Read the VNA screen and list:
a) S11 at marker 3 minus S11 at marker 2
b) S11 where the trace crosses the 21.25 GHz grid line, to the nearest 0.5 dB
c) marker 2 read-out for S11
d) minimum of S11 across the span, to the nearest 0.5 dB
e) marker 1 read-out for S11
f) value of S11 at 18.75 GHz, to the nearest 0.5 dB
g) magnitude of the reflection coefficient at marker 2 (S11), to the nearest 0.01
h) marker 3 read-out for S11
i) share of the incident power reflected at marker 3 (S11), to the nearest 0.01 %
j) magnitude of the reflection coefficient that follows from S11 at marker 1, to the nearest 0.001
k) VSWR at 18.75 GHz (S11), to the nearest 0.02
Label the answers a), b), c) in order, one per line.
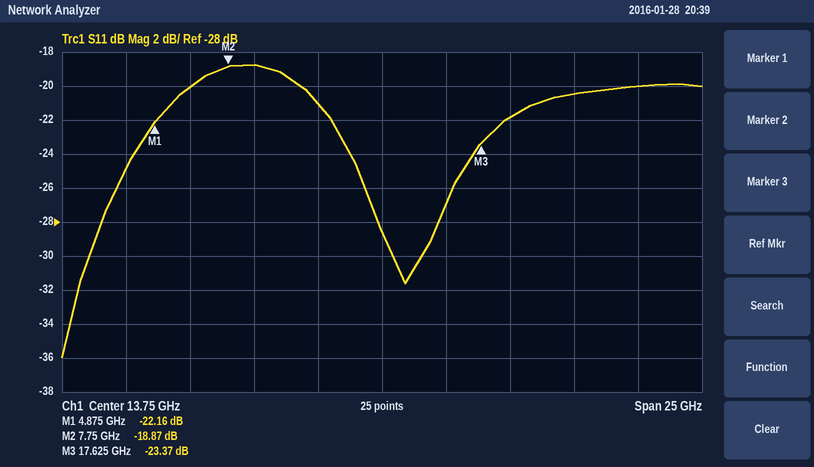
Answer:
a) -4.50 dB
b) -20.5 dB
c) -18.87 dB
d) -36.0 dB
e) -22.16 dB
f) -22.0 dB
g) 0.11
h) -23.37 dB
i) 0.46 %
j) 0.078
k) 1.18
